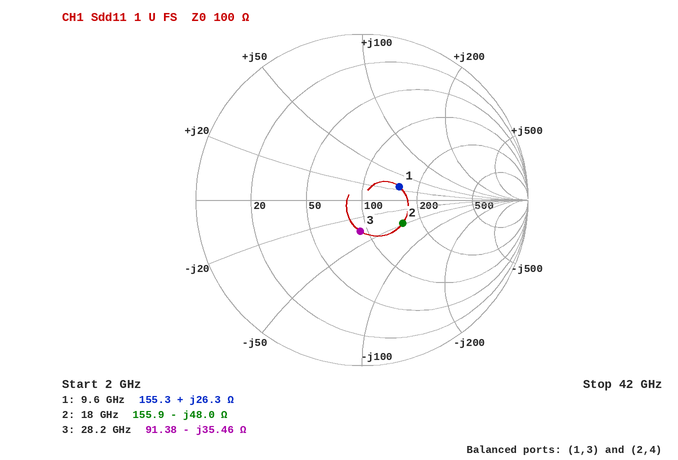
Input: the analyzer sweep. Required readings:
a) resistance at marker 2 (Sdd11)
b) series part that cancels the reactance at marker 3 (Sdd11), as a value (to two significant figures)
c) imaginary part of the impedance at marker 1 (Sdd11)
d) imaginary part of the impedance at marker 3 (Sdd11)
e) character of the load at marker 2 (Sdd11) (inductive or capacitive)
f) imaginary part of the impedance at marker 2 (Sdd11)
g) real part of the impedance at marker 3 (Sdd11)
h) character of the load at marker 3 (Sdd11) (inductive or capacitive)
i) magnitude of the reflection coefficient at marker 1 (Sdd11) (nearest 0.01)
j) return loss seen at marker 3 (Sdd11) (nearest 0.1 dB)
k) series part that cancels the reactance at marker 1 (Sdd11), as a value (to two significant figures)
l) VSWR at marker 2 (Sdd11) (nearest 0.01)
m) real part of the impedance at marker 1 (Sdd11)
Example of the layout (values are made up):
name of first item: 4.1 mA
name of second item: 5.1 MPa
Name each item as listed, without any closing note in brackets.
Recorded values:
resistance at marker 2: 155.9 Ω
series part that cancels the reactance at marker 3 (Sdd11), as a value: 200 pH
imaginary part of the impedance at marker 1: +26.3 Ω
imaginary part of the impedance at marker 3: -35.46 Ω
character of the load at marker 2 (Sdd11): capacitive
imaginary part of the impedance at marker 2: -48.0 Ω
real part of the impedance at marker 3: 91.38 Ω
character of the load at marker 3 (Sdd11): capacitive
magnitude of the reflection coefficient at marker 1 (Sdd11): 0.24
return loss seen at marker 3 (Sdd11): 14.5 dB
series part that cancels the reactance at marker 1 (Sdd11), as a value: 630 fF
VSWR at marker 2 (Sdd11): 1.79
real part of the impedance at marker 1: 155.3 Ω
